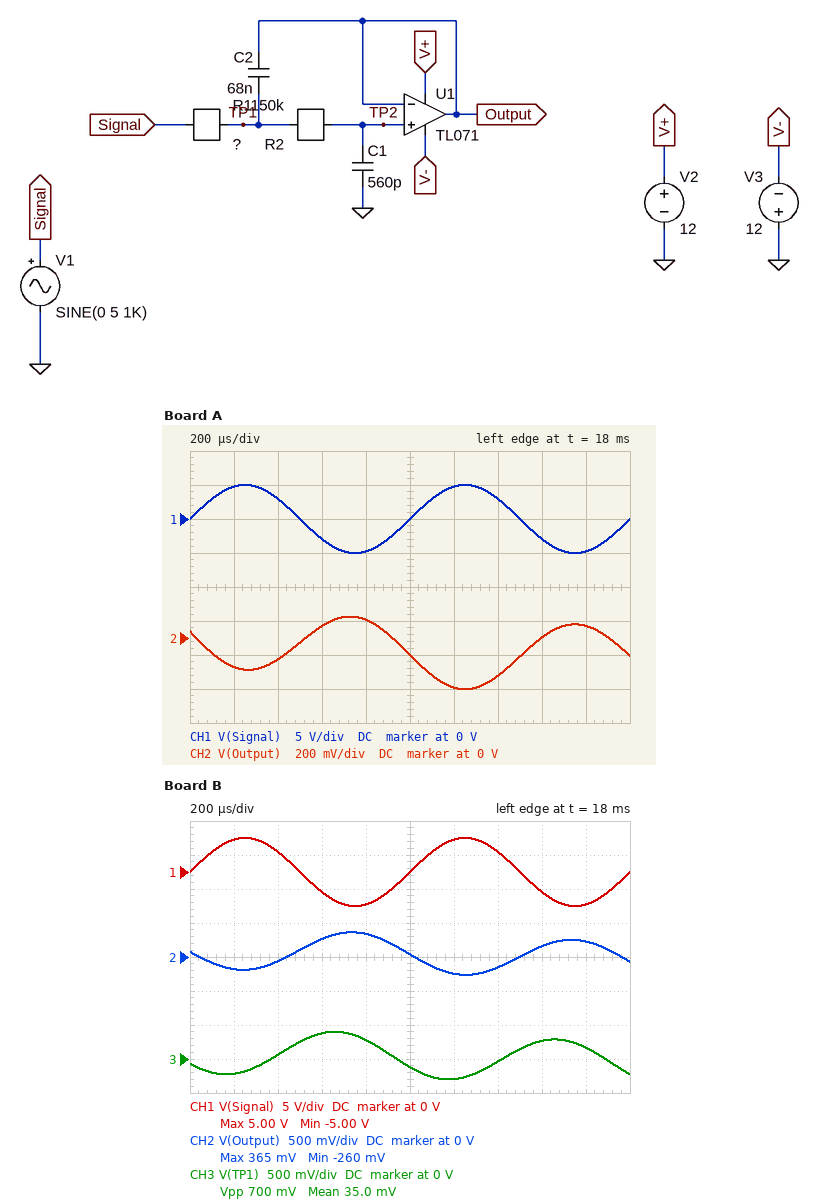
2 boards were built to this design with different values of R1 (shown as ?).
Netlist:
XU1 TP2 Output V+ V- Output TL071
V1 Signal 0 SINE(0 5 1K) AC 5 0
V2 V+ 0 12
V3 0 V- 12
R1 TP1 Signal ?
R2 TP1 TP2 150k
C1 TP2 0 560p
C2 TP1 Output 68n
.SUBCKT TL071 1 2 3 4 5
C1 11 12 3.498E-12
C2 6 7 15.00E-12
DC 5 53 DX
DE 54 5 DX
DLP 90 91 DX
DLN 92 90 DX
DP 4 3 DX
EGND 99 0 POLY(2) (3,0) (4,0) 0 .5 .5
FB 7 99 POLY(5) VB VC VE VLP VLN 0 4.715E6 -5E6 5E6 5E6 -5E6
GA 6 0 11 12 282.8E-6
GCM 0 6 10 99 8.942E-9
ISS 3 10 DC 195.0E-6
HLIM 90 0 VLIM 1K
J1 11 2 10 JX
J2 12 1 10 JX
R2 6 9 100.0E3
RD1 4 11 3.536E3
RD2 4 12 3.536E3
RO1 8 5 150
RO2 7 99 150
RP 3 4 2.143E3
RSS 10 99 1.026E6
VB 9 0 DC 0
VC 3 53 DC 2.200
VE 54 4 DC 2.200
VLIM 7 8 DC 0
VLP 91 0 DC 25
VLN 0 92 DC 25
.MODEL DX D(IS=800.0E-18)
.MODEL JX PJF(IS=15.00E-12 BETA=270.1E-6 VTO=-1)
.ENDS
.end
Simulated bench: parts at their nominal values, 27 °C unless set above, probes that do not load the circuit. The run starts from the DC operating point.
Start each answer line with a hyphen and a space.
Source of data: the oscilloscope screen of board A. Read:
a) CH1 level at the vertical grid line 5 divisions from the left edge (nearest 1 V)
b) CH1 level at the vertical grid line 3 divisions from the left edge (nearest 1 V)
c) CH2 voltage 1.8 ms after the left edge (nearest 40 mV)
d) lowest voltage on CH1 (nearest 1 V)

- 0 V
- -3 V
- 80 mV
- -5 V
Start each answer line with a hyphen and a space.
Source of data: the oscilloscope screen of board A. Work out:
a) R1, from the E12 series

- 120 kΩ
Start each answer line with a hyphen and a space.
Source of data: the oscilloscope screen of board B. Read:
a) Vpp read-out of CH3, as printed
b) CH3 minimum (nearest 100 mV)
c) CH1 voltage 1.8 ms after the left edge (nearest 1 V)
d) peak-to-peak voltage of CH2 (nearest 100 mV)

- 700 mV
- -300 mV
- -5 V
- 600 mV
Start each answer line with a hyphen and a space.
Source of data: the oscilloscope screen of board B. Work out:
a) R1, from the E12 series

- 82 kΩ
